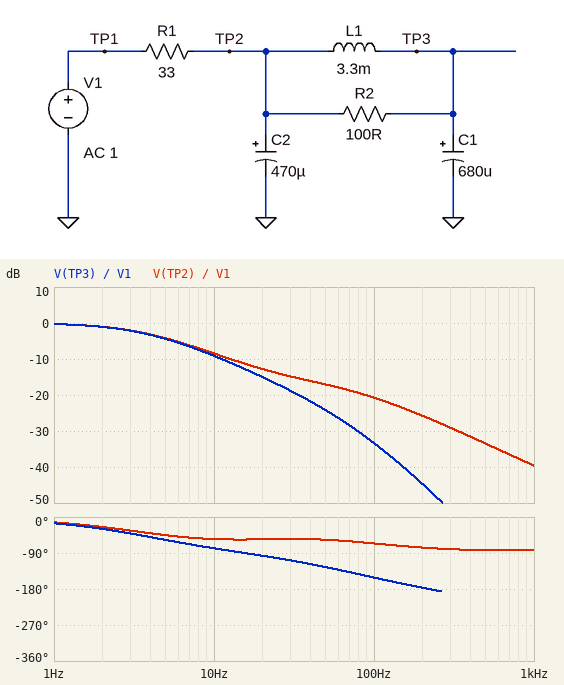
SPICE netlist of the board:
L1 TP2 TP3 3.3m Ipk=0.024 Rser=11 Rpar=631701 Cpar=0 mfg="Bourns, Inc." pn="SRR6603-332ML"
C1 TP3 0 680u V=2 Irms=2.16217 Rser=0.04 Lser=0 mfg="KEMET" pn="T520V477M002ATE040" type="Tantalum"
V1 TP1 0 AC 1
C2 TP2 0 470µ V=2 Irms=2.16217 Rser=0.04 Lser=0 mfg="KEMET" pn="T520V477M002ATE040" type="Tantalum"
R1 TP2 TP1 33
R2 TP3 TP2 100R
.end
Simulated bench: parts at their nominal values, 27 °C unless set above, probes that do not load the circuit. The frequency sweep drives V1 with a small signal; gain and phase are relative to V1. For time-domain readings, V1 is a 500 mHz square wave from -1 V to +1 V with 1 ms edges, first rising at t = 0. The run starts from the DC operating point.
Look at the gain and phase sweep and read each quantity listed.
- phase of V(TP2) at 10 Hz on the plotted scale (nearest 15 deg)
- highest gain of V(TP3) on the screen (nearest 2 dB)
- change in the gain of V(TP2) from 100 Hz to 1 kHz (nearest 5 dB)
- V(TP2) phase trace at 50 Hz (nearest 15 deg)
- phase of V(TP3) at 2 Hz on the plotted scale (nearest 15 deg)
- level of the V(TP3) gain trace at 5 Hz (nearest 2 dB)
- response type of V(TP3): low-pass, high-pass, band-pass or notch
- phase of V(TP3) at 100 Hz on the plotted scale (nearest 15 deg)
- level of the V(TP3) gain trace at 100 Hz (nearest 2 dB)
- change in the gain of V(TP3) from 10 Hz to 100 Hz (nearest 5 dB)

-60 deg
0 dB
-20 dB
-60 deg
-30 deg
-4 dB
low-pass
-150 deg
-34 dB
-25 dB
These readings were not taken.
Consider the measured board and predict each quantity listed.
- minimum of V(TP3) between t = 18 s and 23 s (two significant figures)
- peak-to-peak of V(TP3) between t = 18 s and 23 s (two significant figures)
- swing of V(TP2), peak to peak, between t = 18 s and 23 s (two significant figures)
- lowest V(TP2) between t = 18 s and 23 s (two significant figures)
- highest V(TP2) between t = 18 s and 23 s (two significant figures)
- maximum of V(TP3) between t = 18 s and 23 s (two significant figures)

-1.0 V
2.0 V
2.0 V
-1.0 V
1.0 V
1.0 V
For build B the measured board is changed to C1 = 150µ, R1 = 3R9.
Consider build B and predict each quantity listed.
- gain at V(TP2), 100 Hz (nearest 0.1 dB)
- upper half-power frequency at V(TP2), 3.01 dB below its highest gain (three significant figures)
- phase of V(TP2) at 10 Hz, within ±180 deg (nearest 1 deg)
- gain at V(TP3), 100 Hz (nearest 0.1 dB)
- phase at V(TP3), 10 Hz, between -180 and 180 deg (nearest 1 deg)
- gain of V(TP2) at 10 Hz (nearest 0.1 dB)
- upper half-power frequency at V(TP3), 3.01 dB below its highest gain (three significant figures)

-5.2 dB
60.9 Hz
-9 deg
-7.2 dB
-14 deg
-0.1 dB
51.5 Hz
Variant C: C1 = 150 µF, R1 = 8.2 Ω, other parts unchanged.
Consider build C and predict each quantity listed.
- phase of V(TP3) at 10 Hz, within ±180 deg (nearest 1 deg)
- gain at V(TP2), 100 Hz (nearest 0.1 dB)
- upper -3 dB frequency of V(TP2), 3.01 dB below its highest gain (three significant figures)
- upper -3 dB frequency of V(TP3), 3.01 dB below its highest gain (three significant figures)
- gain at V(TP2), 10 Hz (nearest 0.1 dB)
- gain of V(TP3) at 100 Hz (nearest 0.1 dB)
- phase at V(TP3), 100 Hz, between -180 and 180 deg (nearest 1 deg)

-23 deg
-10.1 dB
29.6 Hz
28.3 Hz
-0.5 dB
-12.1 dB
-110 deg
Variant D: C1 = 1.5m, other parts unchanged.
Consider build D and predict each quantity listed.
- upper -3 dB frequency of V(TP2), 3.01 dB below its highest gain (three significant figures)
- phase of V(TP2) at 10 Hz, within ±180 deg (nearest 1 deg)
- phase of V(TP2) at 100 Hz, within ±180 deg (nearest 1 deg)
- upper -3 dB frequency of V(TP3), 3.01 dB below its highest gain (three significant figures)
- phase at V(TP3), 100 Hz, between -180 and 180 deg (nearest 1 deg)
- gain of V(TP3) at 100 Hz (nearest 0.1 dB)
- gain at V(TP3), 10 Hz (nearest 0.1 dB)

2.15 Hz
-46 deg
-65 deg
2.07 Hz
-157 deg
-39.9 dB
-14.0 dB
